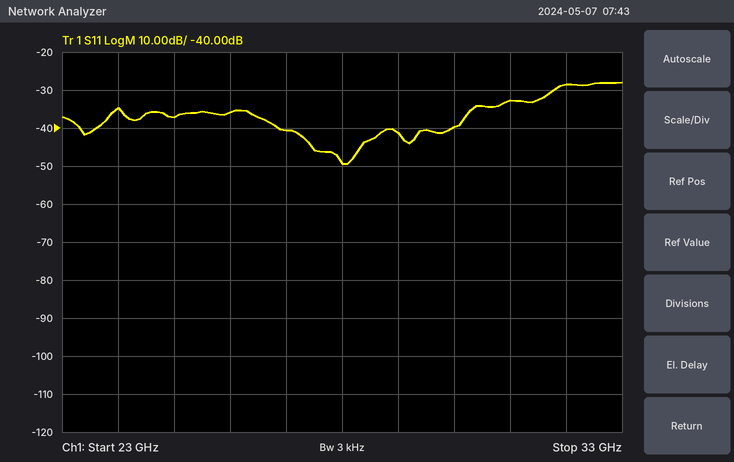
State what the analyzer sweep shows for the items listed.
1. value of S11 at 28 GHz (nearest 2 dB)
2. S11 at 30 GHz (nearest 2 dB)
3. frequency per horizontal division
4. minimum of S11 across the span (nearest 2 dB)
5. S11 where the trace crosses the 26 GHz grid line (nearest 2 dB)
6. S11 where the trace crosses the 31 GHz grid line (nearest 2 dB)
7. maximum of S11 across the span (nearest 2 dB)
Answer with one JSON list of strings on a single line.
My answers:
["-50 dB", "-40 dB", "1 GHz", "-50 dB", "-36 dB", "-32 dB", "-28 dB"]
